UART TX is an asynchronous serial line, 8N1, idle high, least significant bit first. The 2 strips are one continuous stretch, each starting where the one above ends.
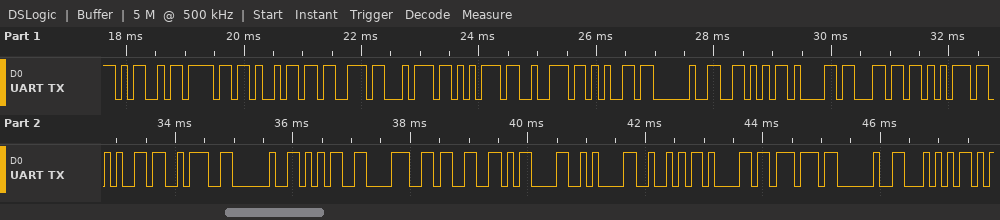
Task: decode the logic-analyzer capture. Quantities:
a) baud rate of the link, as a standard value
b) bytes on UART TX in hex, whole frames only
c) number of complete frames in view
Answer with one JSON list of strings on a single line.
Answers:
["9600 baud", "4D 6F 69 73 74 75 72 65 20 56 61 6C 75 65 3A 20 35 38 33 0D 0A 52 61 77 20 54", "26"]
